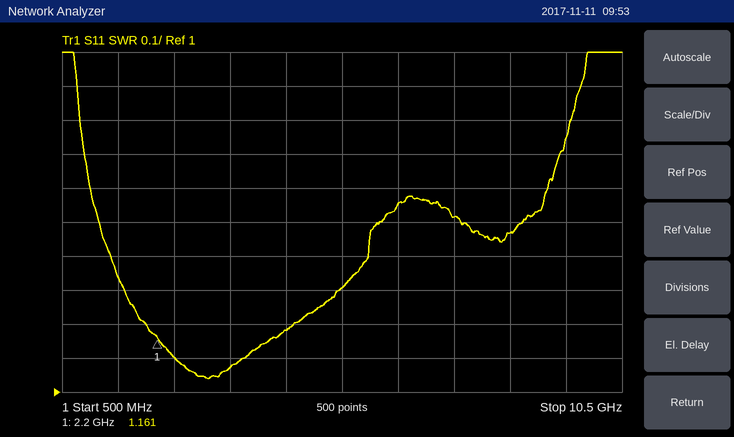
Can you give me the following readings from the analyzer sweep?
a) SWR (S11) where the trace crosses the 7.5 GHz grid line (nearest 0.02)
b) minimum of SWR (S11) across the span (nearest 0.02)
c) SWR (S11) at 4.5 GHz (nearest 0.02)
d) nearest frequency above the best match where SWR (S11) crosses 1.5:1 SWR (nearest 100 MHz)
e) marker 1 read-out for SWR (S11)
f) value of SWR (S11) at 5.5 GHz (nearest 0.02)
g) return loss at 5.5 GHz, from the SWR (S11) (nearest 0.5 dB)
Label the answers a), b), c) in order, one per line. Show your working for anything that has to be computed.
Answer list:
a) 1.52
b) 1.04
c) 1.18
d) 6.2 GHz
e) 1.161
f) 1.30
g) −20 log10((1.3 − 1)/(1.3 + 1)) ≈ 17.7 dB, so 17.5 dB to the nearest 0.5 dB
